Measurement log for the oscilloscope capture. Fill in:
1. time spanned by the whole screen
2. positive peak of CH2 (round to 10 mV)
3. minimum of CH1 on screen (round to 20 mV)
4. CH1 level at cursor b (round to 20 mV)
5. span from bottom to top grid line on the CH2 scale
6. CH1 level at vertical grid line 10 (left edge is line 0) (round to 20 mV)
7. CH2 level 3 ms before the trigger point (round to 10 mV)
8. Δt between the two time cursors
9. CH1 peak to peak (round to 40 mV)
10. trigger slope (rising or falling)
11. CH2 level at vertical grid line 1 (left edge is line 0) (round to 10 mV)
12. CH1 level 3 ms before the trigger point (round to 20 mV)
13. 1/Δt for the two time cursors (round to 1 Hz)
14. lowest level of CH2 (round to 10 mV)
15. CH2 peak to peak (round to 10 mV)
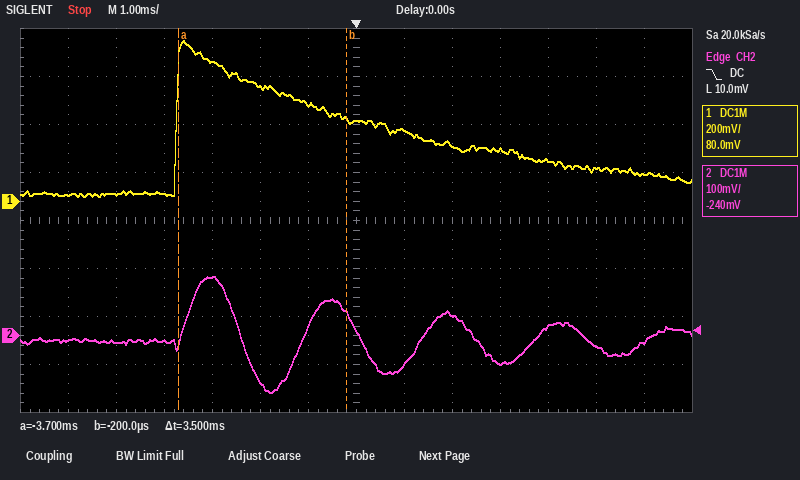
14 ms
120 mV
20 mV
340 mV
800 mV
220 mV
120 mV
3.5 ms
640 mV
falling
-10 mV
580 mV
286 Hz
-120 mV
240 mV
